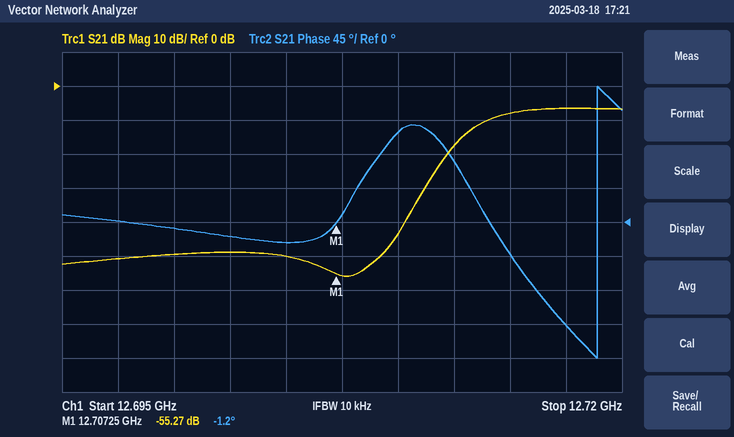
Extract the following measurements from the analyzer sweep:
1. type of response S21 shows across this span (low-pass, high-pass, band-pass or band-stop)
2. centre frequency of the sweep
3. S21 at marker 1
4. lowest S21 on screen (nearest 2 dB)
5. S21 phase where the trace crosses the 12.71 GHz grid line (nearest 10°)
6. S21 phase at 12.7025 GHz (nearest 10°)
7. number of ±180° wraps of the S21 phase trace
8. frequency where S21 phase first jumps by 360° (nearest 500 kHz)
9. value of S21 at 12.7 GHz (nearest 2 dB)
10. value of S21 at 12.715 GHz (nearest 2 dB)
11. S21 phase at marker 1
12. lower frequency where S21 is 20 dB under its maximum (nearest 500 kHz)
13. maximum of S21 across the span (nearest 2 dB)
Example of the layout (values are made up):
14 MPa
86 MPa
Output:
high-pass
12.7075 GHz
-55.27 dB
-56 dB
120°
-20°
1
12.7190 GHz
-50 dB
-8 dB
-1.2°
12.7115 GHz
-6 dB
